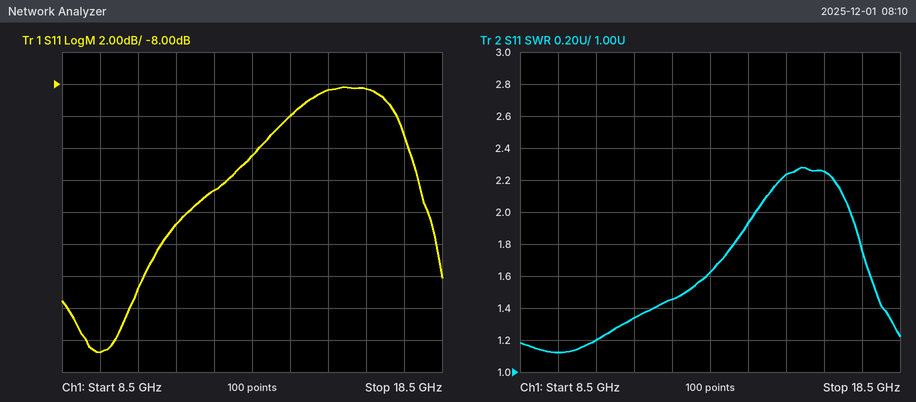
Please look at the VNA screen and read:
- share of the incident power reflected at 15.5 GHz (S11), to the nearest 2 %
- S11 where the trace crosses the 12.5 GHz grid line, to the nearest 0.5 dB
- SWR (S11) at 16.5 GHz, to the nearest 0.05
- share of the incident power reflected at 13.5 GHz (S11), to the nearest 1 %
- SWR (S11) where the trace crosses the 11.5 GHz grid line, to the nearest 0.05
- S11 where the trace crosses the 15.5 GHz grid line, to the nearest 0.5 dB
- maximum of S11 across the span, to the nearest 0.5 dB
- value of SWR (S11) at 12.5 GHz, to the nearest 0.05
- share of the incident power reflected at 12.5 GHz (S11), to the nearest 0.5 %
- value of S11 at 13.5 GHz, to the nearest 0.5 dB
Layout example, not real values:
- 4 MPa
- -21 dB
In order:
- 14 %
- -14.5 dB
- 2.25
- 6 %
- 1.35
- -8.5 dB
- -8.0 dB
- 1.45
- 3.5 %
- -12.5 dB
